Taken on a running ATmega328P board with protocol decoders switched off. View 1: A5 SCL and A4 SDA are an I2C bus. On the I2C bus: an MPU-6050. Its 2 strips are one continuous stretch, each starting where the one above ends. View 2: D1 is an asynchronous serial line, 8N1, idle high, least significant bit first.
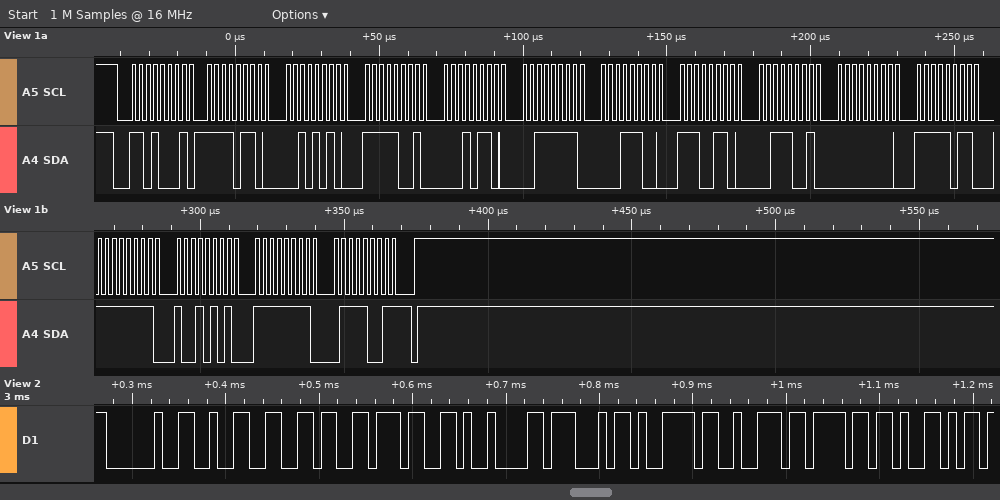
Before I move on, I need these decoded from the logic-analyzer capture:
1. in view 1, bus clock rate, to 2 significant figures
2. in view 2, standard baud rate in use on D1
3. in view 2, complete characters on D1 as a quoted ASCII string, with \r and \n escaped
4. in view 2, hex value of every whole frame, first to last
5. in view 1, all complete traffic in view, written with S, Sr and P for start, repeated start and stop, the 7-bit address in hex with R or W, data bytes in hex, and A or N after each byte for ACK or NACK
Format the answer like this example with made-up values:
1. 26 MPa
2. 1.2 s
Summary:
1. 400 kHz
2. 115200 baud
3. " 267\tGyroY"
4. 20 32 36 37 09 47 79 72 6F 59
5. S 68R A F6 A 2A A F9 A 16 A 3F A 1C A E6 A 39 A 00 A FB A FF A 95 A FF A 79 N P
